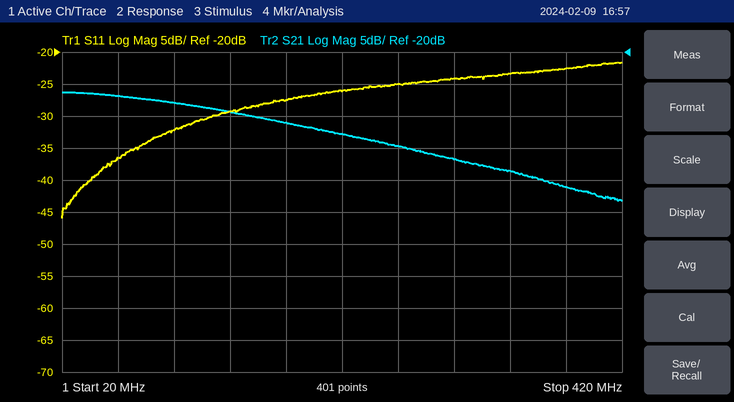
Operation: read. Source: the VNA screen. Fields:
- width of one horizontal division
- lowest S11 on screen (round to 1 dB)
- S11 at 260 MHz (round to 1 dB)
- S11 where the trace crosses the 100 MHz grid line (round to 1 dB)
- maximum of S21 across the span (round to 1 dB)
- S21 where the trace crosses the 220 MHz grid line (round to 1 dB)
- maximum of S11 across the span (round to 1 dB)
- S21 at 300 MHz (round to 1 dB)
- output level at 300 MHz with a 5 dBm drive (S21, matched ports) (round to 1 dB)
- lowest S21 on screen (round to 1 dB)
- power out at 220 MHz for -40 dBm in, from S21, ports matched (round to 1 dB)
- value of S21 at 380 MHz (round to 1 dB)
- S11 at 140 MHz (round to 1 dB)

40 MHz
-46 dB
-25 dB
-32 dB
-26 dB
-33 dB
-22 dB
-37 dB
-32 dBm
-43 dB
-73 dBm
-41 dB
-29 dB
